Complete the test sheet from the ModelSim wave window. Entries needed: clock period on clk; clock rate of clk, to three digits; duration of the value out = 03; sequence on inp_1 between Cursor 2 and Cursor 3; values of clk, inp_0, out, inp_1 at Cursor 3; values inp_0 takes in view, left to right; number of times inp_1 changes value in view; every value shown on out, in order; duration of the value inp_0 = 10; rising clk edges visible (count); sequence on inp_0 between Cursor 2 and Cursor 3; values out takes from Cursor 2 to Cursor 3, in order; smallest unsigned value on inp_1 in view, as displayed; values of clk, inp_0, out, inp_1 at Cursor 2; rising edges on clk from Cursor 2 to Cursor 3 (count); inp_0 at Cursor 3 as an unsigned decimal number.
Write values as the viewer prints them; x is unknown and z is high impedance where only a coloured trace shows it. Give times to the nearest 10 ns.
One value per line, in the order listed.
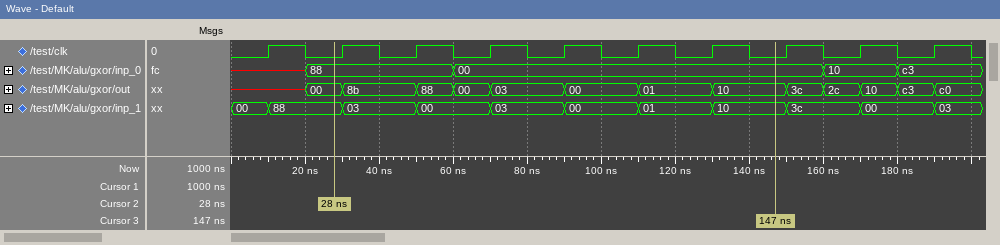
20 ns
50.0 MHz
20 ns
88, 03, 00, 03, 00, 01, 10
clk=0, inp_0=00, out=10, inp_1=10
x, 88, 00, 10, c3
10
x, 00, 8b, 88, 00, 03, 00, 01, 10, 3c, 2c, 10, c3, c0
20 ns
10
88, 00
00, 8b, 88, 00, 03, 00, 01, 10
00
clk=0, inp_0=88, out=00, inp_1=88
6
0
